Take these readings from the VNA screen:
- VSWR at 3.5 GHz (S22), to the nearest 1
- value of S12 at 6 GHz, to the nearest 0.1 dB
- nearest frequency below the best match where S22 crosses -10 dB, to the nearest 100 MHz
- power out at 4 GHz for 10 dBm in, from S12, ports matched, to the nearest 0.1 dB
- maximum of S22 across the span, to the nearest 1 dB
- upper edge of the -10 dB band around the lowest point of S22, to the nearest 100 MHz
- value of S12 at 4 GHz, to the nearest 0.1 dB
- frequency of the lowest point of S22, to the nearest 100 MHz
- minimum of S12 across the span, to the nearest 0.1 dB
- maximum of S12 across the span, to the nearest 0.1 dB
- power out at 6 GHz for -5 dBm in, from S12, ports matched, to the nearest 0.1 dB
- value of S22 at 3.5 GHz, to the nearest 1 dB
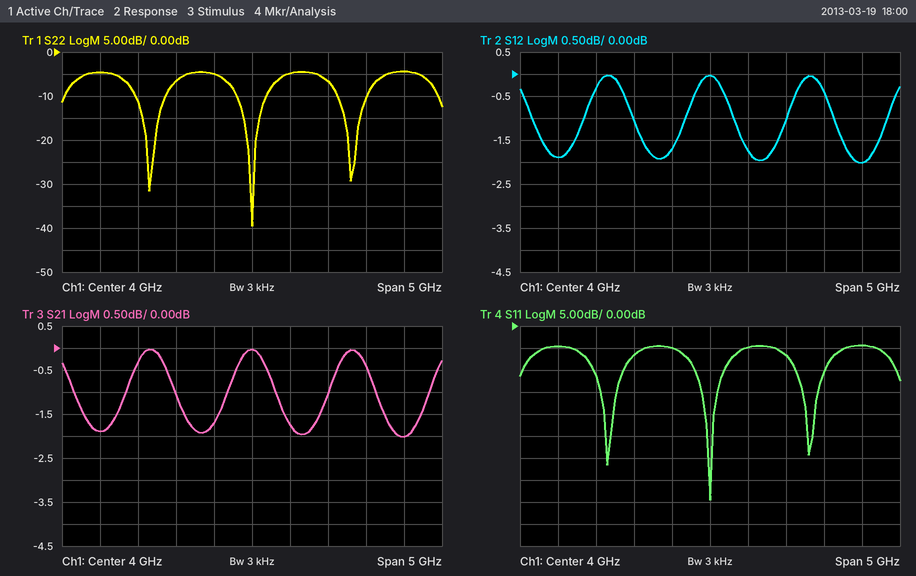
4
-2.0 dB
3.8 GHz
10.0 dBm
-4 dB
4.2 GHz
0.0 dB
4.0 GHz
-2.0 dB
0.0 dB
-7.0 dBm
-5 dB
